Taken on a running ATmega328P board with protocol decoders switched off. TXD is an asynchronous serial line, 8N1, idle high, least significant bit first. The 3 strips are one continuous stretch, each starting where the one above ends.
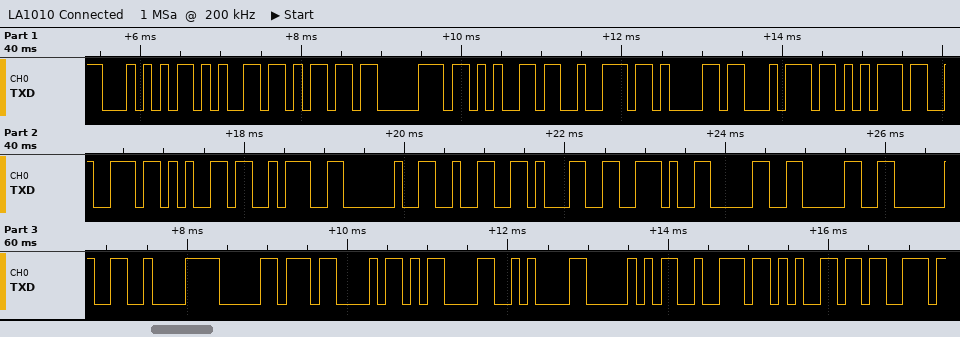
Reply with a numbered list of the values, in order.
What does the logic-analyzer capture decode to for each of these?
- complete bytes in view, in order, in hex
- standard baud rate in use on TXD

1. 54 65 6D 70 65 72 61 74 75 72 65 3A 20 32 31 2E 30 30 20 C2 B0 43 0D 0A 50 72 65 73
2. 9600 baud
